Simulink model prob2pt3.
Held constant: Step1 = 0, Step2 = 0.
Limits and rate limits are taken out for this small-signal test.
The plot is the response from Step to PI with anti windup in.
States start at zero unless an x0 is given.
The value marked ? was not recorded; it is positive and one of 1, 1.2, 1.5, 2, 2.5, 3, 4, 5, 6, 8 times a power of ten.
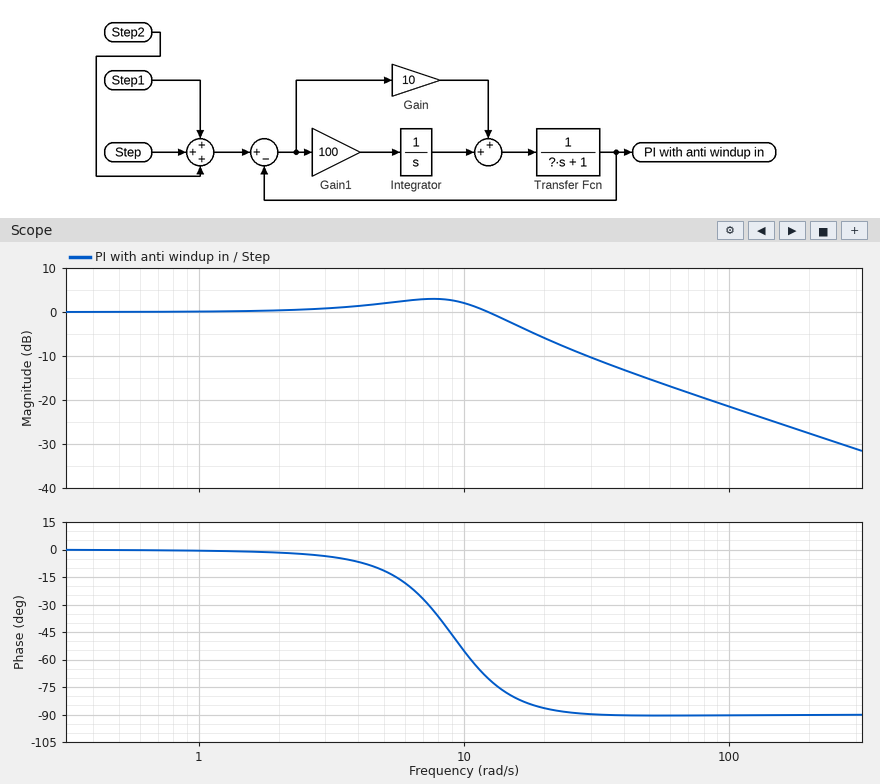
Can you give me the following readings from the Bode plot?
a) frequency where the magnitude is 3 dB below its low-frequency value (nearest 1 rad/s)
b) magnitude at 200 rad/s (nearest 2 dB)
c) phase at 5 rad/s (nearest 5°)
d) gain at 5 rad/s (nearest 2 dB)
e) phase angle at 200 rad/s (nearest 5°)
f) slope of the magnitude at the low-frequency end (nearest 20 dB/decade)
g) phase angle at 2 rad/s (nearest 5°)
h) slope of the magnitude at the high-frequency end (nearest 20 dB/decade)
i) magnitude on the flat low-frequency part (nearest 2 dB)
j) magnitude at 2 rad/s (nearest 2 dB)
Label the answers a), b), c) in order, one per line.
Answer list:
a) 16 rad/s
b) -28 dB
c) -10°
d) 2 dB
e) -90°
f) 0 dB/decade
g) 0°
h) -20 dB/decade
i) 0 dB
j) 0 dB
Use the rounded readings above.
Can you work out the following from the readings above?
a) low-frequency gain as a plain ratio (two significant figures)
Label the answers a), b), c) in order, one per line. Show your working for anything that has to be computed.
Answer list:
a) 10^(0 / 20) = 1.0
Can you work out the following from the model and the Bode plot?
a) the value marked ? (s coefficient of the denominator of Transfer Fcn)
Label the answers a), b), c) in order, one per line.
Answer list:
a) 1.2
